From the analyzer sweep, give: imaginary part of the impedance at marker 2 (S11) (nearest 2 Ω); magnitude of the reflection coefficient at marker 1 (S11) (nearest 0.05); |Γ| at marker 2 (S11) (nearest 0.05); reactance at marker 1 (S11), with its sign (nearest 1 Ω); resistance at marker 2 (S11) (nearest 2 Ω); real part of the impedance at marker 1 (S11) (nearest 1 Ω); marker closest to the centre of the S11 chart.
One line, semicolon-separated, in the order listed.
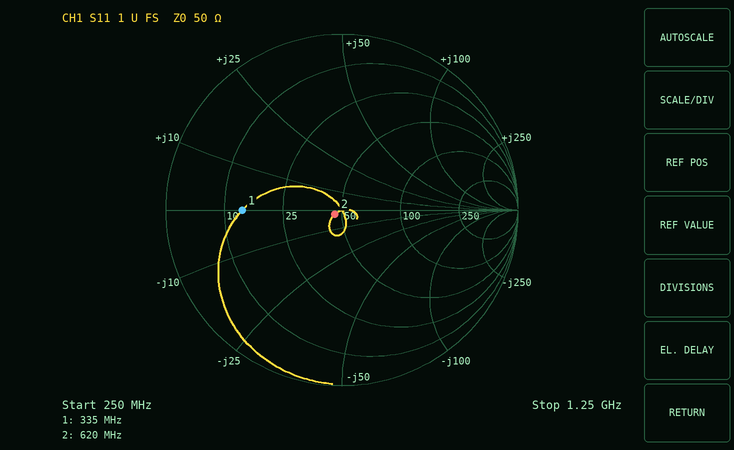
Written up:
-2 Ω; 0.55; 0.05; 0 Ω; 46 Ω; 14 Ω; marker 2
